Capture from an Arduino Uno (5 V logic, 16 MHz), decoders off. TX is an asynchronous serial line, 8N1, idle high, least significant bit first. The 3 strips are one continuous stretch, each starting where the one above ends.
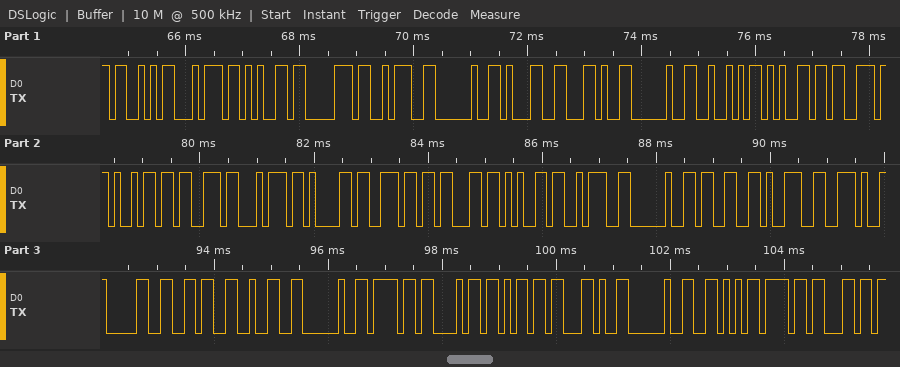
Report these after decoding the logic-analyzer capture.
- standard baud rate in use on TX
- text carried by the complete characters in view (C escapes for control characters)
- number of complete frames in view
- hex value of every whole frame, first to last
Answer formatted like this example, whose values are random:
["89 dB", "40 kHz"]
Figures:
["9600 baud", "\"Step: 1, Resistance: 39.062 ohm, Vol\"", "36", "53 74 65 70 3A 20 31 2C 20 52 65 73 69 73 74 61 6E 63 65 3A 20 33 39 2E 30 36 32 20 6F 68 6D 2C 20 56 6F 6C"]
